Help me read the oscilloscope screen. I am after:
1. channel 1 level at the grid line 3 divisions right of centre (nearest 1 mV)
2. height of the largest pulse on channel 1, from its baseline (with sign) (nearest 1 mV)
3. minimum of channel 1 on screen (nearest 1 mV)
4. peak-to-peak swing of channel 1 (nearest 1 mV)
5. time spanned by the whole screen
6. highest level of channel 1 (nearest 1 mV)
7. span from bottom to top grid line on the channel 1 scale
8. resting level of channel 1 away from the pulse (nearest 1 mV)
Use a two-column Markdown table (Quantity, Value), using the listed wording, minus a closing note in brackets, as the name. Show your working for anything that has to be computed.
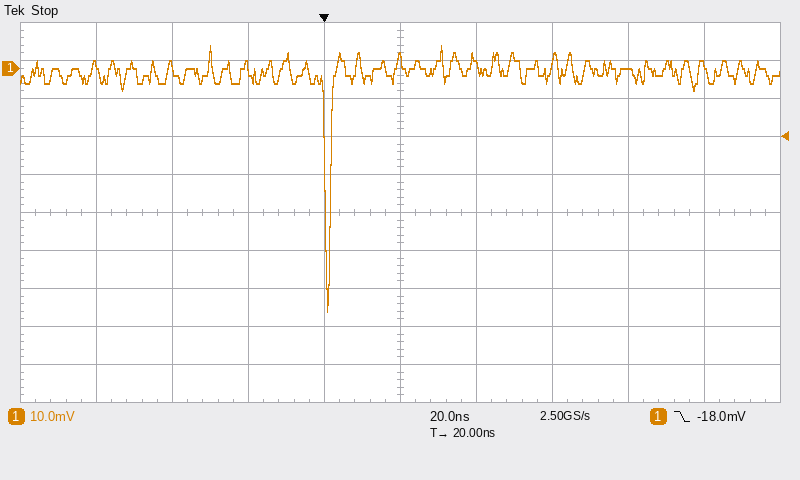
| Quantity | Value |
|---|---|
| channel 1 level at the grid line 3 divisions right of centre | 0 mV |
| height of the largest pulse on channel 1, from its baseline (with sign) | -64 mV − (-1 mV) = -63 mV |
| minimum of channel 1 on screen | -64 mV |
| peak-to-peak swing of channel 1 | 6 mV − (-64 mV) = 70 mV |
| time spanned by the whole screen | 200 ns |
| highest level of channel 1 | 6 mV |
| span from bottom to top grid line on the channel 1 scale | 100 mV |
| resting level of channel 1 away from the pulse | -1 mV |
